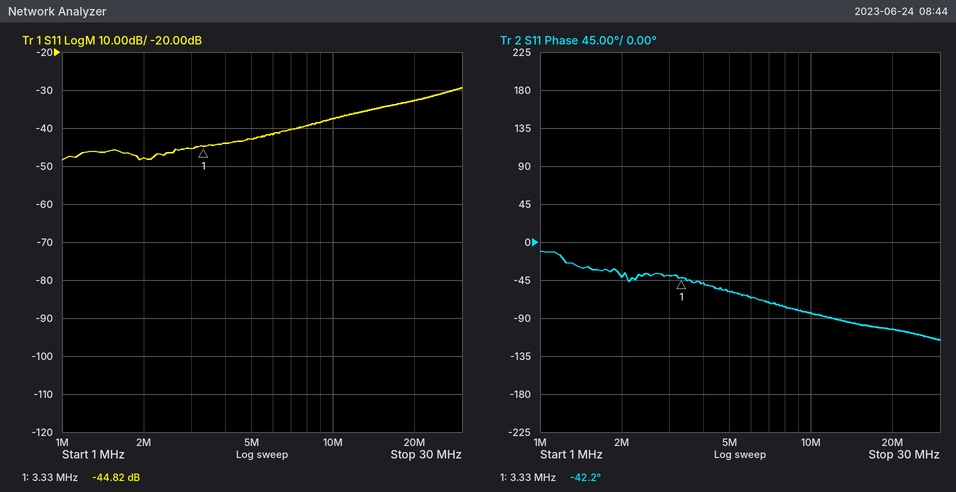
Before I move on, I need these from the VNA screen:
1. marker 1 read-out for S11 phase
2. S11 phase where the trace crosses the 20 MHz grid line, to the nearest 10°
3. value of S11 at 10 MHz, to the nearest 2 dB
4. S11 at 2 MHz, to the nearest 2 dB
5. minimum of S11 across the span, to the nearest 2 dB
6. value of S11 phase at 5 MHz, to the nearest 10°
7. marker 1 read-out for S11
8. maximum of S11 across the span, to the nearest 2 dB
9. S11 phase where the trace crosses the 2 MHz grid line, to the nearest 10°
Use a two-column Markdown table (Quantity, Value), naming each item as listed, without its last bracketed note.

| Quantity | Value |
|---|---|
| marker 1 read-out for S11 phase | -42.2° |
| S11 phase where the trace crosses the 20 MHz grid line, to the nearest 10° | -100° |
| value of S11 at 10 MHz, to the nearest 2 dB | -38 dB |
| S11 at 2 MHz, to the nearest 2 dB | -48 dB |
| minimum of S11 across the span, to the nearest 2 dB | -48 dB |
| value of S11 phase at 5 MHz, to the nearest 10° | -60° |
| marker 1 read-out for S11 | -44.82 dB |
| maximum of S11 across the span, to the nearest 2 dB | -30 dB |
| S11 phase where the trace crosses the 2 MHz grid line, to the nearest 10° | -40° |
